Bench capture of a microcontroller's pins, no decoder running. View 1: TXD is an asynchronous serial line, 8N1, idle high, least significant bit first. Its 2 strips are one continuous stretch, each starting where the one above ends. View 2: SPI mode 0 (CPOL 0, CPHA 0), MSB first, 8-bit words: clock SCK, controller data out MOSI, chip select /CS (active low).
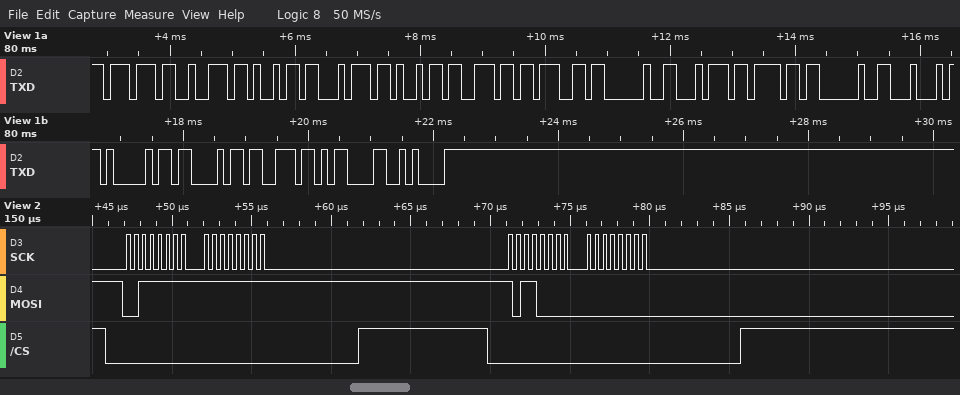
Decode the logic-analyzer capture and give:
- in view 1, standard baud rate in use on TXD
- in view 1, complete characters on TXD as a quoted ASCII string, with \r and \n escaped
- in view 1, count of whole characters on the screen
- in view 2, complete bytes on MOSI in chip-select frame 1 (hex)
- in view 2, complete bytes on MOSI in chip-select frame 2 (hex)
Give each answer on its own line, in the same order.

9600 baud
"writing to DACs\r\n"
17
3F FF
B0 00
